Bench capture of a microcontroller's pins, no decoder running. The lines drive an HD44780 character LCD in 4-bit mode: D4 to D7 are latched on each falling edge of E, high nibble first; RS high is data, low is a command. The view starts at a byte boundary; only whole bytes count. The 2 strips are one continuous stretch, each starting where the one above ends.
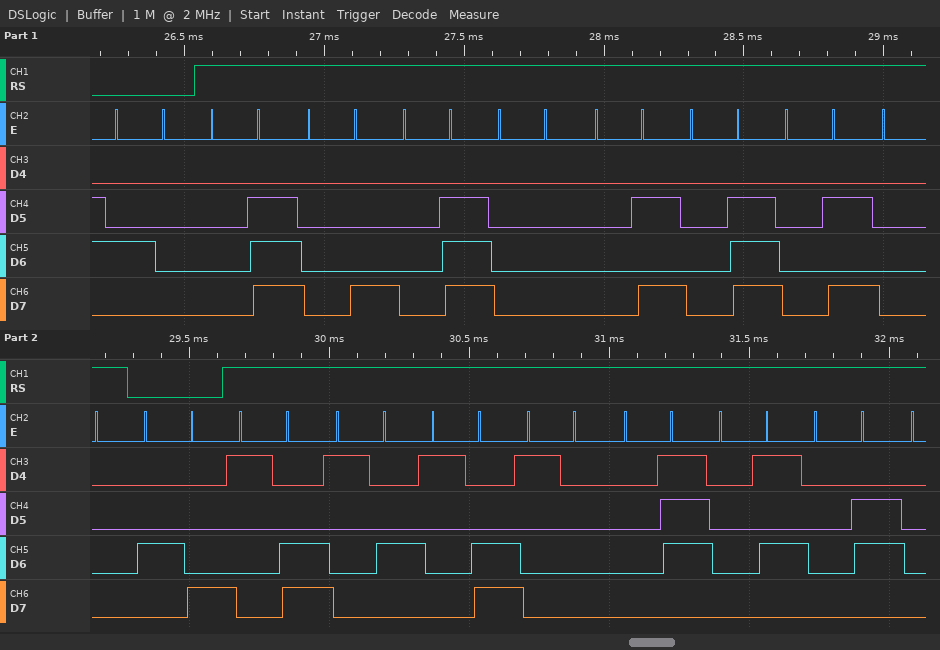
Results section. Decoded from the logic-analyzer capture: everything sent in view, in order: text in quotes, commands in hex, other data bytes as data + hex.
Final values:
0x40 data 0E 08 0E 00 0A 0E 0A 00 0x48 data 1C 14 1C 10 07 05 06
